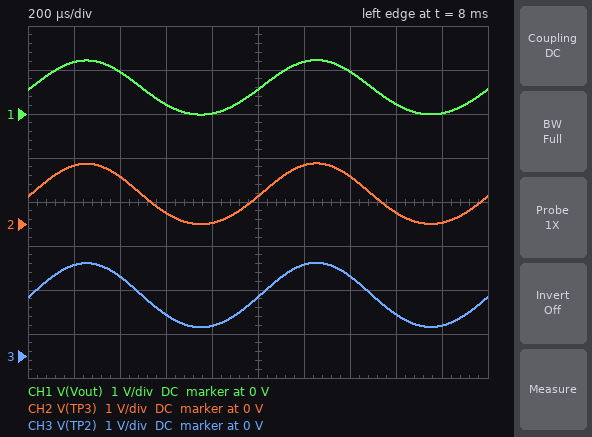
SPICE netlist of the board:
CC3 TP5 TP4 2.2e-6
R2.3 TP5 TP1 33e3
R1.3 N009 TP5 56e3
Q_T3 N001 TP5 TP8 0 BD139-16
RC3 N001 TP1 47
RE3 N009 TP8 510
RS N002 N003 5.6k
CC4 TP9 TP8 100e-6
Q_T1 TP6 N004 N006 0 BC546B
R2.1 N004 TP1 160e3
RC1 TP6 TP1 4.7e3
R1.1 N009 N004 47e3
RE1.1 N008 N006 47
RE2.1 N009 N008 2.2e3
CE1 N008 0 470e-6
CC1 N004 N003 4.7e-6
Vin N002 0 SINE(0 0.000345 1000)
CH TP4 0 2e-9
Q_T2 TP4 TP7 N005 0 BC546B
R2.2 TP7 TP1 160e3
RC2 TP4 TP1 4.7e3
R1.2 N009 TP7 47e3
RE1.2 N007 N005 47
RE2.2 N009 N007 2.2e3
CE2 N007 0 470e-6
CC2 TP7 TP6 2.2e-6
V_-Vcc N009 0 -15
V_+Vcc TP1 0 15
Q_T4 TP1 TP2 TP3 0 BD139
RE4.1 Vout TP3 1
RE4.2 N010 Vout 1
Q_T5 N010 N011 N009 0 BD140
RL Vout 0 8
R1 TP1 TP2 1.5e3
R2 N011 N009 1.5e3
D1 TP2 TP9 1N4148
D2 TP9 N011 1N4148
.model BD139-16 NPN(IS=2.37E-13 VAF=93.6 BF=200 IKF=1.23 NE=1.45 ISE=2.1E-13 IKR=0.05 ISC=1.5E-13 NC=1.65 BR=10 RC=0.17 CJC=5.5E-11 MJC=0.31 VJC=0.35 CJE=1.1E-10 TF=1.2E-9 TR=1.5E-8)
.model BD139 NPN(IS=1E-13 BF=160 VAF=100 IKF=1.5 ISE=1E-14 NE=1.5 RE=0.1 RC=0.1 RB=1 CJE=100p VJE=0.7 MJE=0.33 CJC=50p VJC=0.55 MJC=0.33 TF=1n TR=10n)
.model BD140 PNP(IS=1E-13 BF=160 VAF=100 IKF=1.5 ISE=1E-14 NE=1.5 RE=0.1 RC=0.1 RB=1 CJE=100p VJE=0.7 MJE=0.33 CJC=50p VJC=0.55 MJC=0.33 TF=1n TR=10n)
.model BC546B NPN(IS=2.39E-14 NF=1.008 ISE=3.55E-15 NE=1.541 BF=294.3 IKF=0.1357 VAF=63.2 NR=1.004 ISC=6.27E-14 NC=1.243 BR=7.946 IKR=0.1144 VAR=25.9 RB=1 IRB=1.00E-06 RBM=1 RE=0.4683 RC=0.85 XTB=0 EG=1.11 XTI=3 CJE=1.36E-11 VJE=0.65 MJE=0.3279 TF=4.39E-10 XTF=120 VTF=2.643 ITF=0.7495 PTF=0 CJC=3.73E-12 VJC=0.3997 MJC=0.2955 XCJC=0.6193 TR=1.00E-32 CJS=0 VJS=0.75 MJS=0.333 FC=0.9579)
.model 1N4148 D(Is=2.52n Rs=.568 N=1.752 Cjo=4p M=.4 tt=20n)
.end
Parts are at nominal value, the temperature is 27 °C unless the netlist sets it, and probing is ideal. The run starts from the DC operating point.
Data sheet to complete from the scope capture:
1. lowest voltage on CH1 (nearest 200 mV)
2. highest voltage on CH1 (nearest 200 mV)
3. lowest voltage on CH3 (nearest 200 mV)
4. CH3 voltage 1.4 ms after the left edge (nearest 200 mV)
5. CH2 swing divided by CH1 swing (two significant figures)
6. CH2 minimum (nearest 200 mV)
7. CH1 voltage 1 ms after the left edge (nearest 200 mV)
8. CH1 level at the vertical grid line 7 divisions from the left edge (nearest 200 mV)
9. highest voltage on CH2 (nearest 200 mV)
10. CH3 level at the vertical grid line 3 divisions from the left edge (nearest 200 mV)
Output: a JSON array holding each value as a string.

["0 V", "1.2 V", "600 mV", "1.8 V", "1.1", "0 V", "600 mV", "1.0 V", "1.4 V", "1.0 V"]
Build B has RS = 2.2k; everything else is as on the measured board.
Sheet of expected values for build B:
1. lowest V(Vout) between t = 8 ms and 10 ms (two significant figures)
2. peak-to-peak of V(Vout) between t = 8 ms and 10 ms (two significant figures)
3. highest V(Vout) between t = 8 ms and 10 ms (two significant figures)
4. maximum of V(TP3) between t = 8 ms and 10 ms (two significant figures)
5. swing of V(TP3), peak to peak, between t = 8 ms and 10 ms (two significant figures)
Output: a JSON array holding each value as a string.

["-100 mV", "1.5 V", "1.4 V", "1.6 V", "1.7 V"]
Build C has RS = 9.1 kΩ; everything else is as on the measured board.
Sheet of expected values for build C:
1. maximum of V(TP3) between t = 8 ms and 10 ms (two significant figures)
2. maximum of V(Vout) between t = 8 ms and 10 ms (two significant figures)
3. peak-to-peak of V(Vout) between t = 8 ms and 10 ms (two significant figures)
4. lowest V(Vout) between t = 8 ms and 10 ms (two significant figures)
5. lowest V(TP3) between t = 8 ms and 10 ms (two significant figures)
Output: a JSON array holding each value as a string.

["1.2 V", "1.1 V", "1.0 V", "60 mV", "78 mV"]
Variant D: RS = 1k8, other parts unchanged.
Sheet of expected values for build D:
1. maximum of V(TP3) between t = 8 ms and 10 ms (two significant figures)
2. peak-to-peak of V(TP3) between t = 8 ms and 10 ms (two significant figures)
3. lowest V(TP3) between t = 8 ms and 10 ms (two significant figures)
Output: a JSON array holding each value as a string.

["1.6 V", "1.7 V", "-110 mV"]
